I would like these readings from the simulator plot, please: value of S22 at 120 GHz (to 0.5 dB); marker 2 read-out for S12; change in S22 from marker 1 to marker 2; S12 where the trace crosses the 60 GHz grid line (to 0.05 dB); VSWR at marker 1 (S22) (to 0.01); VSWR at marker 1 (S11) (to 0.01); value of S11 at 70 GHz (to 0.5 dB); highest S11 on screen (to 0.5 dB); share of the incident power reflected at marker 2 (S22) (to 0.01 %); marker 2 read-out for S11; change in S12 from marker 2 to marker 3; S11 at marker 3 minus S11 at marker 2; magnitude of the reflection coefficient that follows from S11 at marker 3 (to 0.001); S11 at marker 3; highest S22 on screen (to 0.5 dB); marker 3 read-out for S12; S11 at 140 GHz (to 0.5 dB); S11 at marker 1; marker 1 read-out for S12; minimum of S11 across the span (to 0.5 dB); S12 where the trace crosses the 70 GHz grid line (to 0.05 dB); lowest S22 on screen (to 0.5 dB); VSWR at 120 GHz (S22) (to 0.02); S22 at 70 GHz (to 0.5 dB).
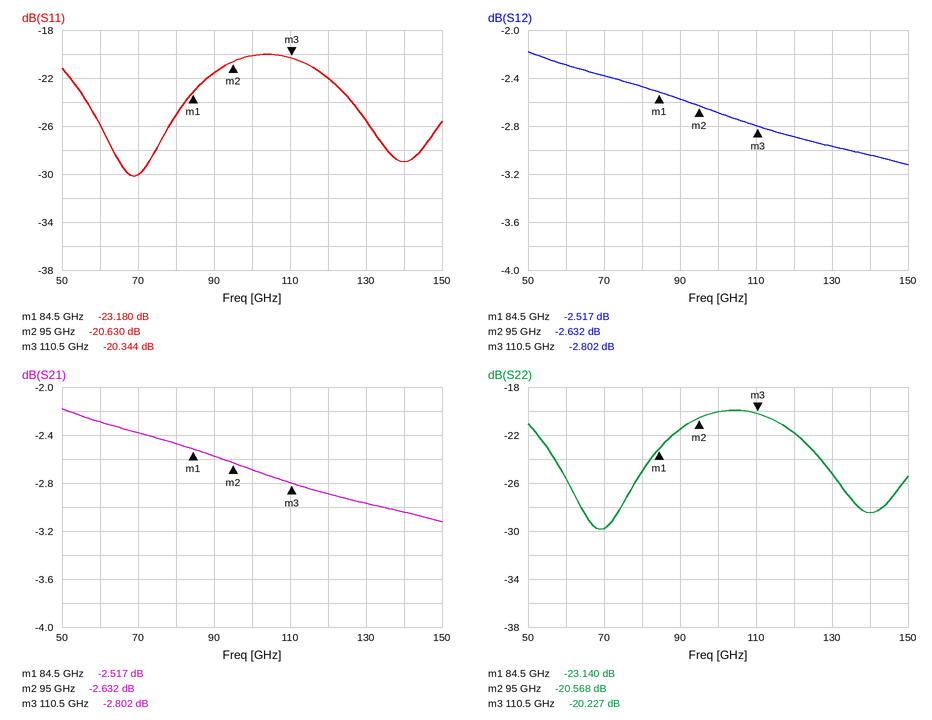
-22.0 dB
-2.632 dB
2.572 dB
-2.30 dB
1.15
1.15
-30.0 dB
-20.0 dB
0.88 %
-20.630 dB
-0.170 dB
0.286 dB
0.096
-20.344 dB
-20.0 dB
-2.802 dB
-29.0 dB
-23.180 dB
-2.517 dB
-30.0 dB
-2.40 dB
-30.0 dB
1.18
-30.0 dB
